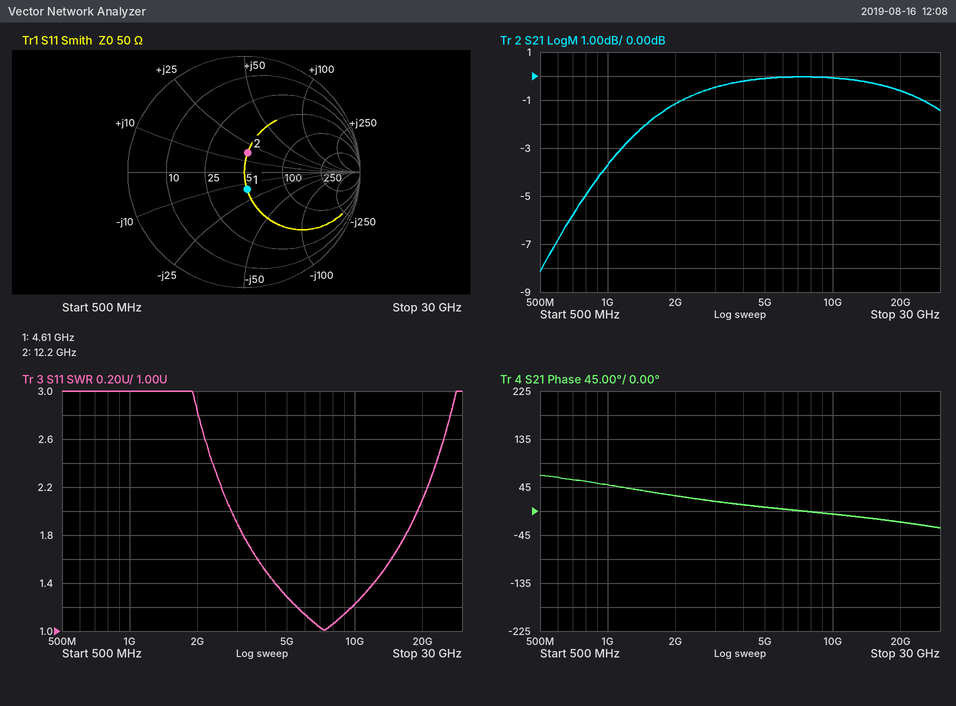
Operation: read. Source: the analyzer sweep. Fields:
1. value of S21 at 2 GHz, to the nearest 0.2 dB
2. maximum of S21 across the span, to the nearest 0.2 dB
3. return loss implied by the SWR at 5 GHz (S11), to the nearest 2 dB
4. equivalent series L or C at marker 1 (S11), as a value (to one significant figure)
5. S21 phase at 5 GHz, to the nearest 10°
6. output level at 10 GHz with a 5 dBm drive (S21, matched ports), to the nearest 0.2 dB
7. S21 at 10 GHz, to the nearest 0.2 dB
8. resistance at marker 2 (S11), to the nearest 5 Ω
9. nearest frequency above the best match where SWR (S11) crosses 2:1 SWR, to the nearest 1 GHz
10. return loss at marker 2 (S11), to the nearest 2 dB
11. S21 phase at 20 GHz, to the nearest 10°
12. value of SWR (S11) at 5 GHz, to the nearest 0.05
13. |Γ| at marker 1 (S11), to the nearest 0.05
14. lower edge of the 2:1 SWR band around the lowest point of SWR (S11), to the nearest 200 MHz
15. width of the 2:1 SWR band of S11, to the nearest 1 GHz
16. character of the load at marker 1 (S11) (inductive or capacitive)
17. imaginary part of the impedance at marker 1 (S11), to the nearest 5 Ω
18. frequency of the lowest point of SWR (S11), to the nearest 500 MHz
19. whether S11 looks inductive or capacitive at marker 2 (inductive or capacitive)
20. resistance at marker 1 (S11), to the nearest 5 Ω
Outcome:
-1.2 dB
0.0 dB
18 dB
2 pF
10°
5.0 dBm
0.0 dB
50 Ω
19 GHz
16 dB
-20°
1.30
0.15
2.8 GHz
16 GHz
capacitive
-15 Ω
7.5 GHz
inductive
50 Ω
